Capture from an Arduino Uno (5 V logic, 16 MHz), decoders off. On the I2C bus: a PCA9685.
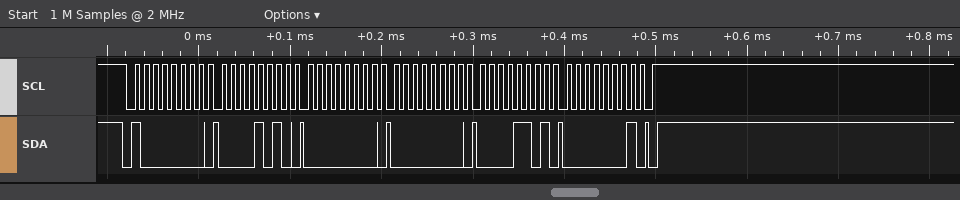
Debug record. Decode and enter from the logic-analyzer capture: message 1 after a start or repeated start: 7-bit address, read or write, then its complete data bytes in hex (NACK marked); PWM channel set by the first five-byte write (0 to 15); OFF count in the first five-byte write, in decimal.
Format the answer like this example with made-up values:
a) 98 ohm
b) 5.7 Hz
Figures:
a) 0x40 write: 0A 00 00 0D 01
b) 1
c) 269
